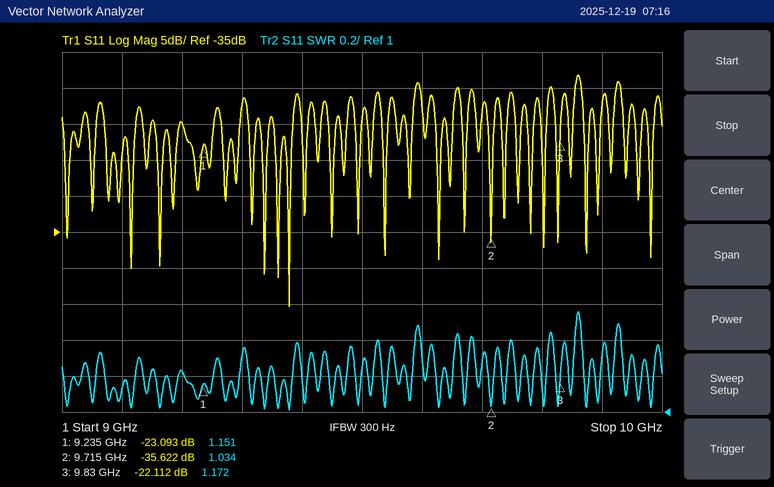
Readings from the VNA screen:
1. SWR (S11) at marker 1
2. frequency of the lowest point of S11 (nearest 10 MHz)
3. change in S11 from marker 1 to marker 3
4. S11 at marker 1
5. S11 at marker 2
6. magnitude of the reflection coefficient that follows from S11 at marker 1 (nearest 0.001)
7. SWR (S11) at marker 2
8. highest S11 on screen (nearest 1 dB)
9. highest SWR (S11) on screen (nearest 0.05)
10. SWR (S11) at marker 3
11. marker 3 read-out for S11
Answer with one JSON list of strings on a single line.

["1.151", "9.38 GHz", "0.981 dB", "-23.093 dB", "-35.622 dB", "0.070", "1.034", "-13 dB", "1.55", "1.172", "-22.112 dB"]
